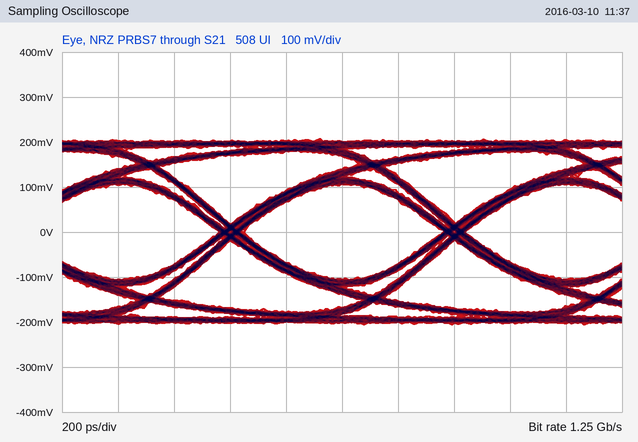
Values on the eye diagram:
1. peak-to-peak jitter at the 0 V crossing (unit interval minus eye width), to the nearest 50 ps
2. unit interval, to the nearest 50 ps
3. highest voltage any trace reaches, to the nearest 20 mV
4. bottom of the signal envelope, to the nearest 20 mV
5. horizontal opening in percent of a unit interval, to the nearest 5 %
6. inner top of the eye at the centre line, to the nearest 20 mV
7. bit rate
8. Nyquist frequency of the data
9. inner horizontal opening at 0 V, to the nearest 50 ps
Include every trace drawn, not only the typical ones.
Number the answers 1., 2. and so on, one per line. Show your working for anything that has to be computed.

1. 100 ps
2. 800 ps
3. 200 mV
4. -200 mV
5. 700 ps / 800 ps ≈ 87.5 %, so 90 % to the nearest 5 %
6. 100 mV
7. 1.25 Gb/s
8. 625 MHz
9. 700 ps
